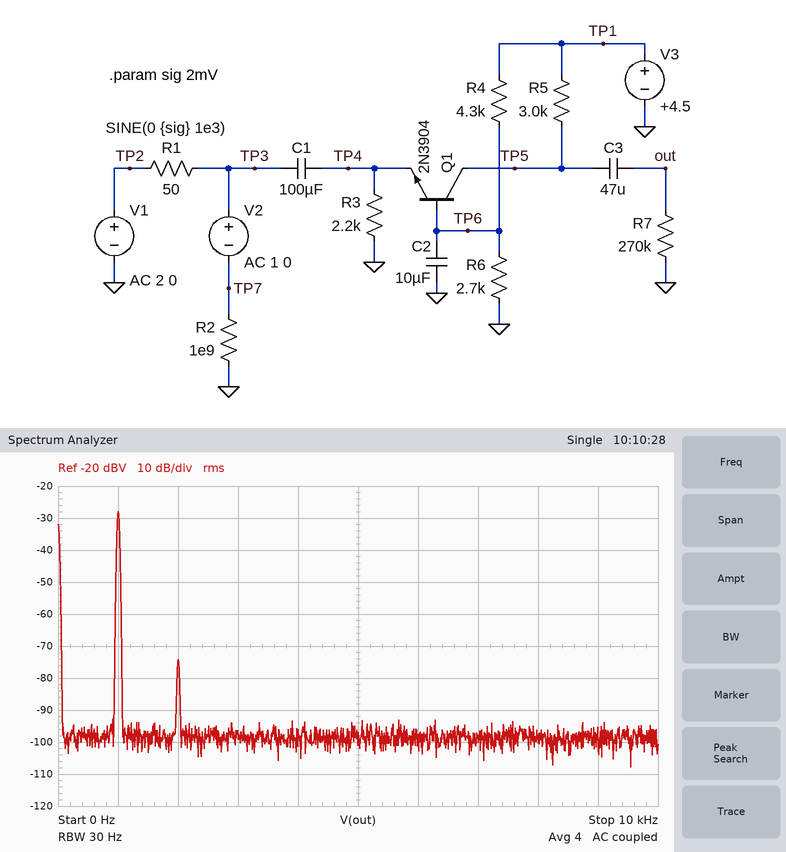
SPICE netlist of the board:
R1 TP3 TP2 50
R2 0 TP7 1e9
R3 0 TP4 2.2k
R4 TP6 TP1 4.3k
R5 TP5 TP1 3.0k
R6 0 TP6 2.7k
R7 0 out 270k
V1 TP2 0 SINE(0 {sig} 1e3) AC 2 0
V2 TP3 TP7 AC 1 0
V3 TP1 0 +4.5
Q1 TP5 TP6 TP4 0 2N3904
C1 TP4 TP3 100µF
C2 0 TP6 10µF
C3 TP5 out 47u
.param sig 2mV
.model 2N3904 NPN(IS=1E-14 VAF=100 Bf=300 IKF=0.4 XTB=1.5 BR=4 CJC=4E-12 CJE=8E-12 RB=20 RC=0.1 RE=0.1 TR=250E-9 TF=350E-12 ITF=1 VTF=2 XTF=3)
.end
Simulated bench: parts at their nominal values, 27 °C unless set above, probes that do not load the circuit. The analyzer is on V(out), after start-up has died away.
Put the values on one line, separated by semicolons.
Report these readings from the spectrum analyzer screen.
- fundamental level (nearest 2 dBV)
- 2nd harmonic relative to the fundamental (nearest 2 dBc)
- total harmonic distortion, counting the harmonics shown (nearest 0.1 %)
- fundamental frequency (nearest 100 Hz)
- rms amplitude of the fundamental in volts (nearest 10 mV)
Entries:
-28 dBV; -46 dBc; 0.5 %; 1.0 kHz; 40 mV
